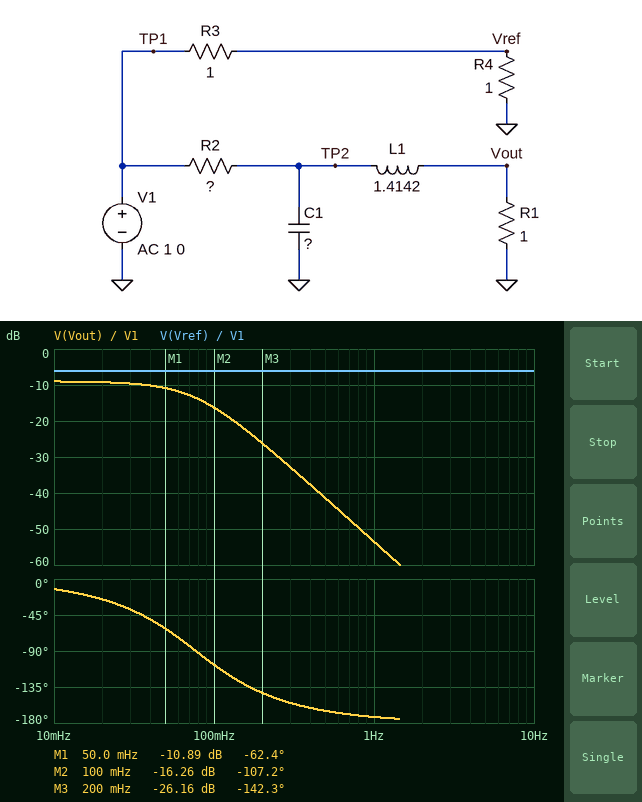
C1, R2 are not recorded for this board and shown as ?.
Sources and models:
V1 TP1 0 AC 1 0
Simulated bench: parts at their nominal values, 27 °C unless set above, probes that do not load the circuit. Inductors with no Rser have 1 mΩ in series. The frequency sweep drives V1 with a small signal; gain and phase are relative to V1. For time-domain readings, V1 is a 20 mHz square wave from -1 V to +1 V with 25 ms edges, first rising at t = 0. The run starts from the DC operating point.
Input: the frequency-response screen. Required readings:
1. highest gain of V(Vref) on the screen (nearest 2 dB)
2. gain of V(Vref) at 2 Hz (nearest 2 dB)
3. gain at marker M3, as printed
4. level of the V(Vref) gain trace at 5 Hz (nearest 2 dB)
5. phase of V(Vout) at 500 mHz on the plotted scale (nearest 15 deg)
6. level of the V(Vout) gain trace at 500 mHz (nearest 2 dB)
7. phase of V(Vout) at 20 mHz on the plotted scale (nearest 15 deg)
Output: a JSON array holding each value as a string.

["-6 dB", "-6 dB", "-26.16 dB", "-6 dB", "-165 deg", "-42 dB", "-30 deg"]
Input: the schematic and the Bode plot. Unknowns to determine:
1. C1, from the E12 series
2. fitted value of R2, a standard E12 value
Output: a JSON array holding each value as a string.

["4.7 F", "1.8 Ω"]
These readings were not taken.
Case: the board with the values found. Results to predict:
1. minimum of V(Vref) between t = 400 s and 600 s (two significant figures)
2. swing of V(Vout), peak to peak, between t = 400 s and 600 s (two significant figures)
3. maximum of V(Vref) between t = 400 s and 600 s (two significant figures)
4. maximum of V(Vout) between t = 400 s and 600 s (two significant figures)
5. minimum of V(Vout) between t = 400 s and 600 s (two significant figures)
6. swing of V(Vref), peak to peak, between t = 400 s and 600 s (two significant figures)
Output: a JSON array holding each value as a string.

["-500 mV", "720 mV", "500 mV", "360 mV", "-360 mV", "1.0 V"]
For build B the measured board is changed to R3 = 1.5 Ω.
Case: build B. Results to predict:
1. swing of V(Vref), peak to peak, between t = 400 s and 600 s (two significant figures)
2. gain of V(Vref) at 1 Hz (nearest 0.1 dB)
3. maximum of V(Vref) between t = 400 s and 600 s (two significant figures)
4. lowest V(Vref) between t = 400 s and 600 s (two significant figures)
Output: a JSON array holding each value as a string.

["800 mV", "-8.0 dB", "400 mV", "-400 mV"]
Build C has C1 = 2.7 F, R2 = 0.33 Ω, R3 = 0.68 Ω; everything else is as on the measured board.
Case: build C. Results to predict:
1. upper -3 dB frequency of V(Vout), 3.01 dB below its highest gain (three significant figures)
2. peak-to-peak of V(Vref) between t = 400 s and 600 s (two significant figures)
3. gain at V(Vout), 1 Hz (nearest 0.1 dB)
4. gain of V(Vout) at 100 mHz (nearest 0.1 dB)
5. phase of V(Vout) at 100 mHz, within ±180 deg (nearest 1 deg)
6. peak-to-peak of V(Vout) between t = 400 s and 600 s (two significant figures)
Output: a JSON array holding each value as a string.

["124 mHz", "1.2 V", "-34.1 dB", "-4.5 dB", "-60 deg", "1.5 V"]
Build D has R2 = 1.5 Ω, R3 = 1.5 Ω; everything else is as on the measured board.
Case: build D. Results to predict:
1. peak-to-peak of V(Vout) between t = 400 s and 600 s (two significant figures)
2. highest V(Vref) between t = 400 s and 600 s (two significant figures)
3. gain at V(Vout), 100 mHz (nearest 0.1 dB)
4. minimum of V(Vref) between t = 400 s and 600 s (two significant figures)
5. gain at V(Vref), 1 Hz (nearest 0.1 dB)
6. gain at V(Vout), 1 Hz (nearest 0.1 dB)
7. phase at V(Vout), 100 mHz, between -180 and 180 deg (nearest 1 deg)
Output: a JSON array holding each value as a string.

["810 mV", "400 mV", "-14.8 dB", "-400 mV", "-8.0 dB", "-51.9 dB", "-105 deg"]
